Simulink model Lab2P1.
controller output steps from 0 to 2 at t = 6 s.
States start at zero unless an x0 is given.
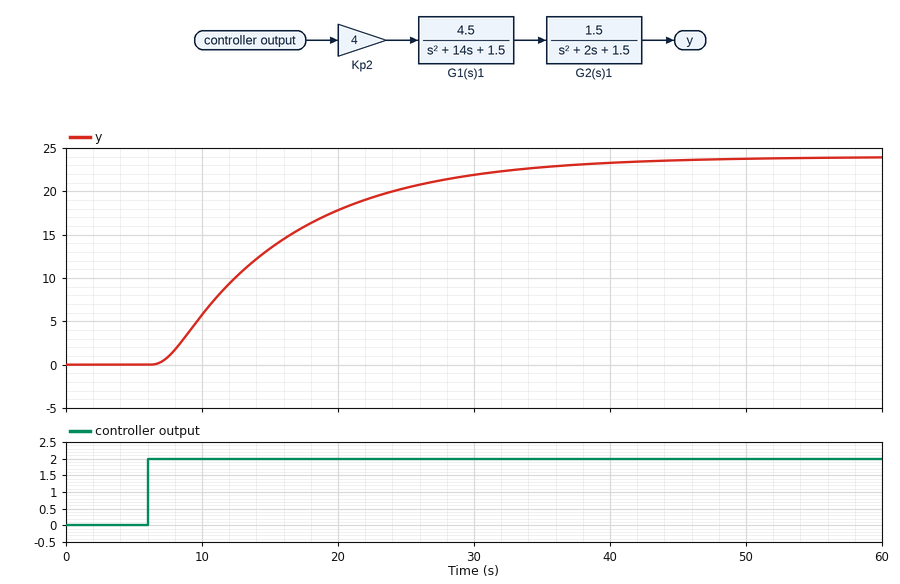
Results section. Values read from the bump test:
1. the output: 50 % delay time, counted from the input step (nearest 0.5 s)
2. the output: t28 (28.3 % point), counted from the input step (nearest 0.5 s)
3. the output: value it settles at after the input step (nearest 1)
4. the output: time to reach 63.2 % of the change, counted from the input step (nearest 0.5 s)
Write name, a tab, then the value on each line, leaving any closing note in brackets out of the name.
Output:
the output: 50 % delay time, counted from the input step	8.0 s
the output: t28 (28.3 % point), counted from the input step	4.5 s
the output: value it settles at after the input step	24
the output: time to reach 63.2 % of the change, counted from the input step	10.5 s
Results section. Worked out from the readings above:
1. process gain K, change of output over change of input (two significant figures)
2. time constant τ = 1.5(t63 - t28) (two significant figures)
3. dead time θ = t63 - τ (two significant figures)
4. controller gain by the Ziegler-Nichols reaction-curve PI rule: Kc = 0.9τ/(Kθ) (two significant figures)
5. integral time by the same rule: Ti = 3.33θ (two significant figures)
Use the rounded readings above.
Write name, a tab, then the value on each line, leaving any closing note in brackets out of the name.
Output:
process gain K, change of output over change of input	12
time constant τ = 1.5(t63 - t28)	9.0 s
dead time θ = t63 - τ	1.5 s
controller gain by the Ziegler-Nichols reaction-curve PI rule: Kc = 0.9τ/(Kθ)	0.45
integral time by the same rule: Ti = 3.33θ	5.0 s
